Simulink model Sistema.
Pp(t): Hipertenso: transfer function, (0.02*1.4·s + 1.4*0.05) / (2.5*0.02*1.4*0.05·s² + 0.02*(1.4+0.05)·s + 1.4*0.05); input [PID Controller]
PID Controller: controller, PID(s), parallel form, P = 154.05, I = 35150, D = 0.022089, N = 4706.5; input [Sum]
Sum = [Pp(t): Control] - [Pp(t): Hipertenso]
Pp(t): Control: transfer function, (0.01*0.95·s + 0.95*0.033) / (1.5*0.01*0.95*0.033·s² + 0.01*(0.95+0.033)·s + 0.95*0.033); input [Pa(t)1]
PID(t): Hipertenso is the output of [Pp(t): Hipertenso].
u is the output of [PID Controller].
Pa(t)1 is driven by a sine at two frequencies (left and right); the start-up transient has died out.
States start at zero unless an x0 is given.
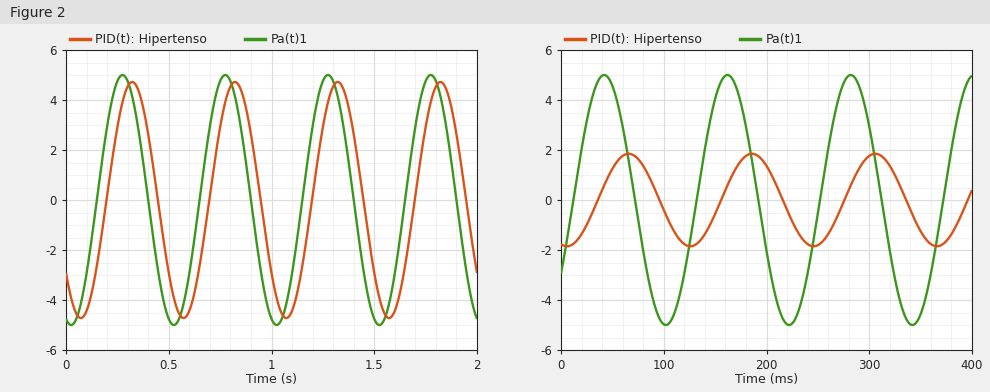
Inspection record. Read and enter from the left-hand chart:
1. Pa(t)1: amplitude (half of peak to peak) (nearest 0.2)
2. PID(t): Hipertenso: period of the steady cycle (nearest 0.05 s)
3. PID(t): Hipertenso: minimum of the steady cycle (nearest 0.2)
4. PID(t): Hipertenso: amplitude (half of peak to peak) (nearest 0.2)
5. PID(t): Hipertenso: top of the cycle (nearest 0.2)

5.0
0.50 s
-4.8
4.8
4.8
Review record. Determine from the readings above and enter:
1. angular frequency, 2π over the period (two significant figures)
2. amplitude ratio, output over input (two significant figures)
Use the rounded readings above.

13 rad/s
0.96
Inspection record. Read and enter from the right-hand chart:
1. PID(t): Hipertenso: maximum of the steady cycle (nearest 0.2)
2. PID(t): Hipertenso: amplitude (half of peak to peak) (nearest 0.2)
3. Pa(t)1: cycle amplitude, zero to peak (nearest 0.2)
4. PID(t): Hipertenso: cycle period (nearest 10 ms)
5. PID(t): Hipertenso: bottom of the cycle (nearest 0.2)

1.8
1.8
5.0
120 ms
-1.8
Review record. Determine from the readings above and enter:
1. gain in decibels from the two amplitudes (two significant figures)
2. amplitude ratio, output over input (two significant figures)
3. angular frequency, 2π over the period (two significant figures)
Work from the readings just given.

-8.9 dB
0.36
0.052 rad/ms
